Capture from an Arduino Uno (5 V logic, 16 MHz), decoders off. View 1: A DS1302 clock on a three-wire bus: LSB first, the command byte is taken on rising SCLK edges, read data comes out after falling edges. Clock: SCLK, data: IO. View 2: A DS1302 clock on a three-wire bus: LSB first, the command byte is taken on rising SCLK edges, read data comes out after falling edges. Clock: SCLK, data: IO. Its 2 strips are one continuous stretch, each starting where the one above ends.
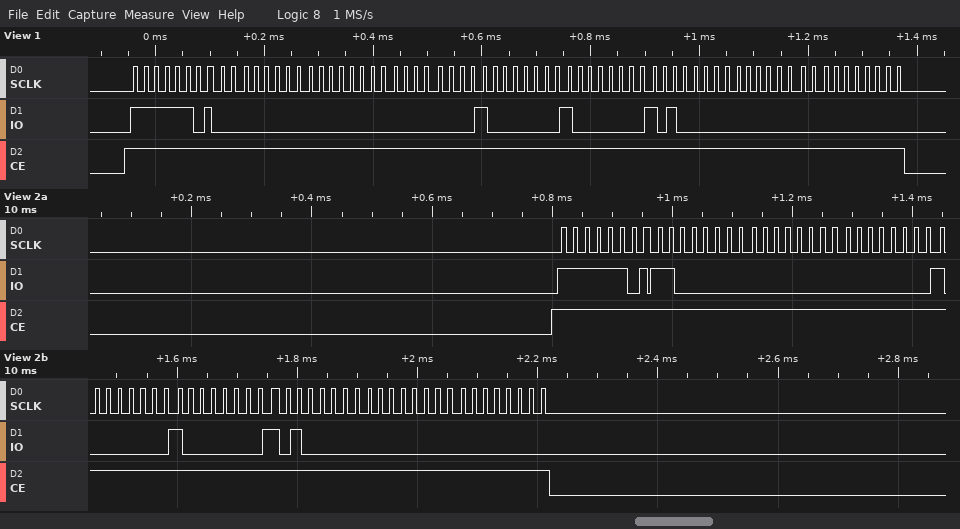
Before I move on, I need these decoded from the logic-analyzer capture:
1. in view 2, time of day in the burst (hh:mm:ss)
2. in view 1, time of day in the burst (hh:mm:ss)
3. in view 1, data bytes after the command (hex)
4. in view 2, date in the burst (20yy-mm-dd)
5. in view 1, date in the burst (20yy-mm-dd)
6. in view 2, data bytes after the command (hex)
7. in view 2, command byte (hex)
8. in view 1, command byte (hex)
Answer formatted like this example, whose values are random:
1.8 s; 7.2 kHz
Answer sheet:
00:00:03; 00:00:00; 00 00 00 01 01 05 00 00; 2000-01-01; 2000-01-01; 03 00 00 01 01 05 00 00; 0xBF; 0xBF
